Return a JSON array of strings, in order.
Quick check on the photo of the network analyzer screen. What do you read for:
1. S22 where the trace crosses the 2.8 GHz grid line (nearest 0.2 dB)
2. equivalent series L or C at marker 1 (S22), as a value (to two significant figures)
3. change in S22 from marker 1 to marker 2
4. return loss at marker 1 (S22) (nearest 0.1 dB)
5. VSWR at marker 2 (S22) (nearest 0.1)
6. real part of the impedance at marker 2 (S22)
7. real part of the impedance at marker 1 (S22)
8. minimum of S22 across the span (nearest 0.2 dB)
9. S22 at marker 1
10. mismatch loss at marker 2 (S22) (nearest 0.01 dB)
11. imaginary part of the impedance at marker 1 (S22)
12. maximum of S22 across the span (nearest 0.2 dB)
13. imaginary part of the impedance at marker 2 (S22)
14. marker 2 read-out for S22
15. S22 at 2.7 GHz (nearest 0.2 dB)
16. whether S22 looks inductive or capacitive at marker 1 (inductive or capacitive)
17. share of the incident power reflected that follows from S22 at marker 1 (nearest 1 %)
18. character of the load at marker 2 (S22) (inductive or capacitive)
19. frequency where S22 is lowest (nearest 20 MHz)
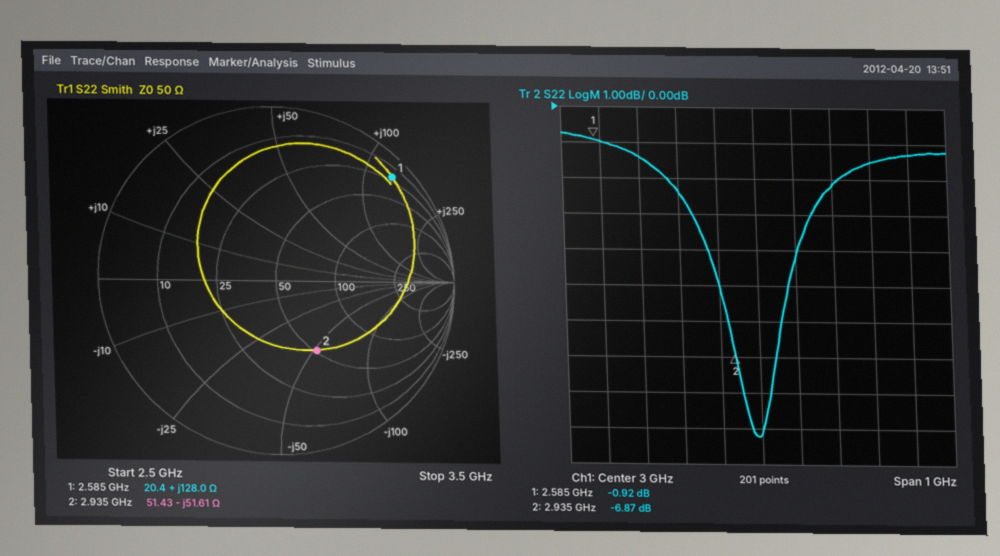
["-2.4 dB", "7.9 nH", "-5.95 dB", "0.9 dB", "2.7", "51.43 Ω", "20.4 Ω", "-9.2 dB", "-0.92 dB", "1.00 dB", "+128.0 Ω", "-0.8 dB", "-51.61 Ω", "-6.87 dB", "-1.4 dB", "inductive", "81 %", "capacitive", "3.00 GHz"]
